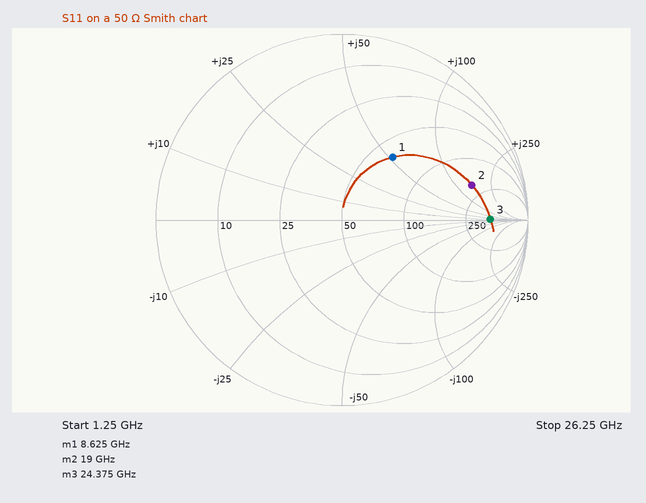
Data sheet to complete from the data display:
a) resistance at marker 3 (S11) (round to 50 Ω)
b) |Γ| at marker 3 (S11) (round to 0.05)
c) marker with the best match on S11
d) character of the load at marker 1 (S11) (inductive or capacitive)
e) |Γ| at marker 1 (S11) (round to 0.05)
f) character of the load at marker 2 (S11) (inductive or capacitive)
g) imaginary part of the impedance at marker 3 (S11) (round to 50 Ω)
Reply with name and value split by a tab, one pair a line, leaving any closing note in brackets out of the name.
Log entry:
resistance at marker 3 (S11)	450 Ω
|Γ| at marker 3 (S11)	0.80
marker with the best match on S11	marker 1
character of the load at marker 1 (S11)	inductive
|Γ| at marker 1 (S11)	0.45
character of the load at marker 2 (S11)	inductive
imaginary part of the impedance at marker 3 (S11)	0 Ω
